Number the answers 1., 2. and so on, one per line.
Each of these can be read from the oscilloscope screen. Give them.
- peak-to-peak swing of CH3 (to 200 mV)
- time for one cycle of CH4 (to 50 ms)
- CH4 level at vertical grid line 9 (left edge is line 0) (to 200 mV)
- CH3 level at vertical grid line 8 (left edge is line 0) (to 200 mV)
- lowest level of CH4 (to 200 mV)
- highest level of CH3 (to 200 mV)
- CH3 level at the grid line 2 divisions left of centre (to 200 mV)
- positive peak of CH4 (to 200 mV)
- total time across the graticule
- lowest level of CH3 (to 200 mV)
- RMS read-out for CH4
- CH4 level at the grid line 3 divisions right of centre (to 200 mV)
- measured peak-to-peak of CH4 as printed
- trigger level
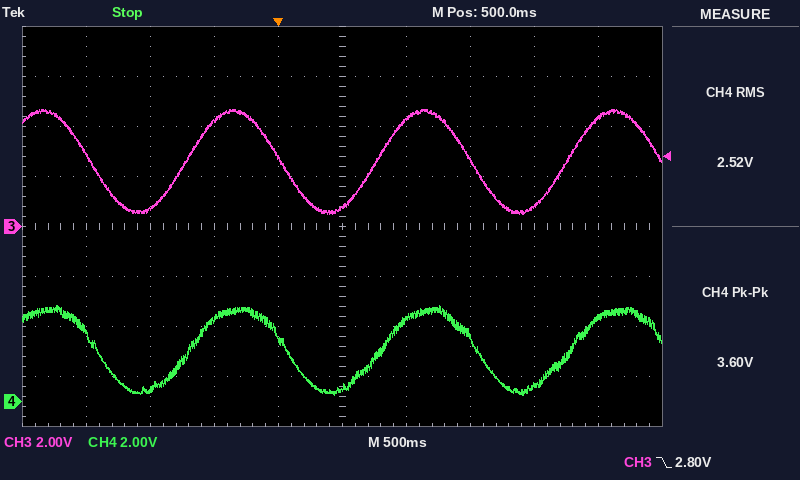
1. 4.2 V
2. 1.50 s
3. 3.4 V
4. 800 mV
5. 200 mV
6. 4.6 V
7. 4.2 V
8. 3.8 V
9. 5 s
10. 400 mV
11. 2.52 V
12. 600 mV
13. 3.60 V
14. 2.80 V
